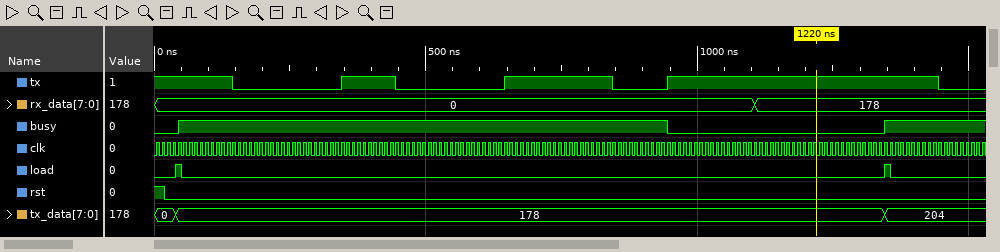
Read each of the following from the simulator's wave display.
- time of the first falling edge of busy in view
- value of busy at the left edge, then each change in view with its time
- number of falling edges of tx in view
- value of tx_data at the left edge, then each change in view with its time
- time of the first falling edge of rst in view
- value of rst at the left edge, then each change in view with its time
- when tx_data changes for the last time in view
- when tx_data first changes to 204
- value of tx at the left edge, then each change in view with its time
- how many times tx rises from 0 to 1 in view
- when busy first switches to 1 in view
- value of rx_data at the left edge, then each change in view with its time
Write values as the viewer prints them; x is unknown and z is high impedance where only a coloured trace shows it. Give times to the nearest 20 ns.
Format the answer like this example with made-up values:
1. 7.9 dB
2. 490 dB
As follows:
1. 940 ns
2. 0, 1 at 40 ns, 0 at 940 ns, 1 at 1340 ns
3. 4
4. 0, 178 at 40 ns, 204 at 1340 ns
5. 20 ns
6. 1, 0 at 20 ns
7. 1340 ns
8. 1340 ns
9. 1, 0 at 140 ns, 1 at 340 ns, 0 at 440 ns, 1 at 640 ns, 0 at 840 ns, 1 at 940 ns, 0 at 1440 ns
10. 3
11. 40 ns
12. 0, 178 at 1100 ns
